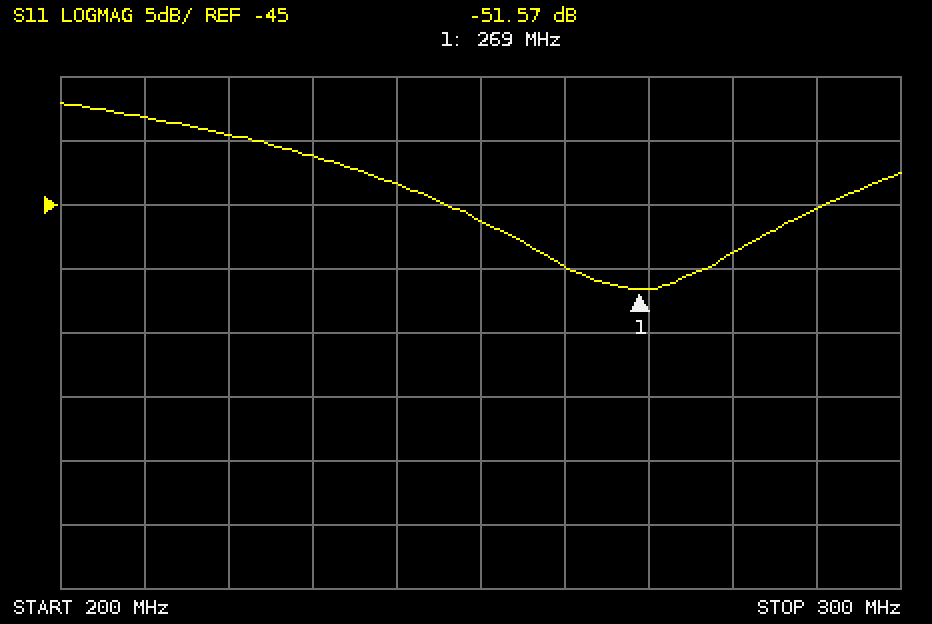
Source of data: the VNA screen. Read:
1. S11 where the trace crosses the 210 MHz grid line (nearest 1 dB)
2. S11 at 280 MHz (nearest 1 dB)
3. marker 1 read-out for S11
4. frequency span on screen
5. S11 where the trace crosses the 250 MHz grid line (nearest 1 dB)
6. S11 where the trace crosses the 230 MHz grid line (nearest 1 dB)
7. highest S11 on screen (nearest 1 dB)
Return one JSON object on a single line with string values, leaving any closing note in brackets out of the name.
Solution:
{"S11 where the trace crosses the 210 MHz grid line": "-38 dB", "S11 at 280 MHz": "-49 dB", "marker 1 read-out for S11": "-51.57 dB", "frequency span on screen": "100 MHz", "S11 where the trace crosses the 250 MHz grid line": "-46 dB", "S11 where the trace crosses the 230 MHz grid line": "-41 dB", "highest S11 on screen": "-37 dB"}
